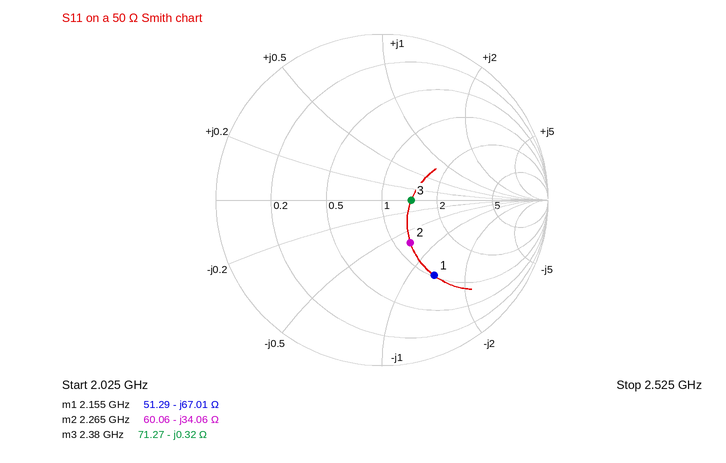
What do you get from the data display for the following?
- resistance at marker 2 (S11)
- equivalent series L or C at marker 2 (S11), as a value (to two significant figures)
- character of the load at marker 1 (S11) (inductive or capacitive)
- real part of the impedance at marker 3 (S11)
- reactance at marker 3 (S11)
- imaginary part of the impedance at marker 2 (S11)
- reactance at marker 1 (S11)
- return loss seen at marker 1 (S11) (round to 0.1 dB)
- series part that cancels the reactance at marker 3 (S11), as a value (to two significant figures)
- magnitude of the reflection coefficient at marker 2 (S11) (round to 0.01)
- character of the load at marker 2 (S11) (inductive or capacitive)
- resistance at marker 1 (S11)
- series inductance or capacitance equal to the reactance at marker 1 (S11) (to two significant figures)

60.06 Ω
2.1 pF
capacitive
71.27 Ω
-0.32 Ω
-34.06 Ω
-67.01 Ω
5.2 dB
21 pH
0.31
capacitive
51.29 Ω
1.1 pF
